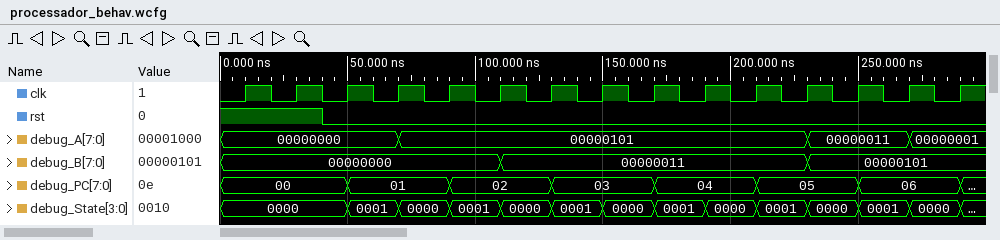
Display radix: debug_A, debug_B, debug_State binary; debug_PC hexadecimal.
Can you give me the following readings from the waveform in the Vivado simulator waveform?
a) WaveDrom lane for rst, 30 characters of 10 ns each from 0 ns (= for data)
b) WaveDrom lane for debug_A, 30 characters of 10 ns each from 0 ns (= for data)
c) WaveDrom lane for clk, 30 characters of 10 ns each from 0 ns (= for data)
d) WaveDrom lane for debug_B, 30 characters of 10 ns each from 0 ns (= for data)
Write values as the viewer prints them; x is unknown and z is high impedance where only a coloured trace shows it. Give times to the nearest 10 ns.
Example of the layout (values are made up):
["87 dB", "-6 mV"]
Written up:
["{name: 'rst', wave: '1...0.........................'}", "{name: 'debug_A', wave: '=......=...............=...=..', data: '00000000 00000101 00000011 00000001'}", "{name: 'clk', wave: '010101010101010101010101010101'}", "{name: 'debug_B', wave: '=..........=...........=......', data: '00000000 00000011 00000101'}"]
